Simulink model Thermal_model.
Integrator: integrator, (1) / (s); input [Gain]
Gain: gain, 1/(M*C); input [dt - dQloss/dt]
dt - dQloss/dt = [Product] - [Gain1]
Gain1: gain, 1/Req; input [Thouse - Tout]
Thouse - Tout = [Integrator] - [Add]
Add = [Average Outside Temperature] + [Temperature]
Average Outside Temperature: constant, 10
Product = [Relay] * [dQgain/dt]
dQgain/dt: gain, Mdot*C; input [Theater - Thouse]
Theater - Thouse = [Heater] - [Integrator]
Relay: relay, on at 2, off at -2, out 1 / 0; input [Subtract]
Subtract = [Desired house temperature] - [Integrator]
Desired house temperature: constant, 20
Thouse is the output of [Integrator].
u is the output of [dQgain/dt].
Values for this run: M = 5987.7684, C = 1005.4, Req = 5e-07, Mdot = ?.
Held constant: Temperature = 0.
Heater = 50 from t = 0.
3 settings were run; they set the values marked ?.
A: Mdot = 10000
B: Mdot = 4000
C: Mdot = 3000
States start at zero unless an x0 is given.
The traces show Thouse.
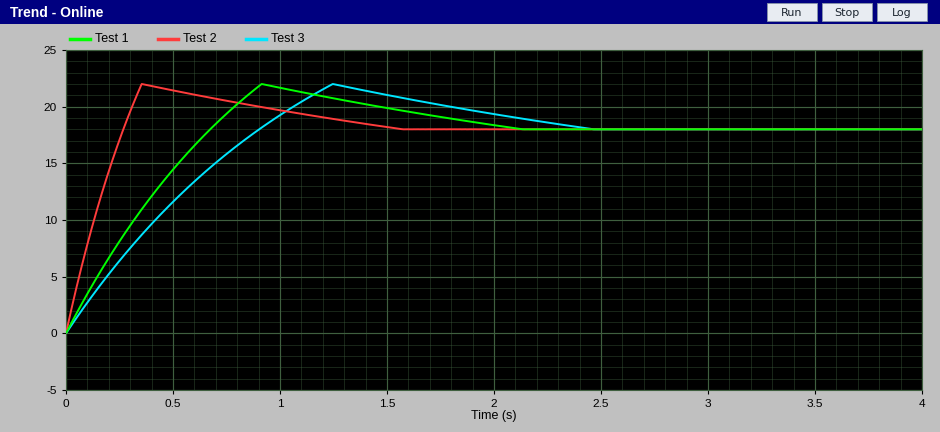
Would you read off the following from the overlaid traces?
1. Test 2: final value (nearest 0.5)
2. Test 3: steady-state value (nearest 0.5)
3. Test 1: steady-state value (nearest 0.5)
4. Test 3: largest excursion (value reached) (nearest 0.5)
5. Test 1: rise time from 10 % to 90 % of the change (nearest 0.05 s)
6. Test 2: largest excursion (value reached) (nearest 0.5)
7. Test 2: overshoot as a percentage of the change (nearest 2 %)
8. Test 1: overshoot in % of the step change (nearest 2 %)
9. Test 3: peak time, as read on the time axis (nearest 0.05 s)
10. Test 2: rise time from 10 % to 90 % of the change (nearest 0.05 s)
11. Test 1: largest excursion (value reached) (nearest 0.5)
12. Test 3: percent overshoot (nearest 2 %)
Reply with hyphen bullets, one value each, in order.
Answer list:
- 18.0
- 18.0
- 18.0
- 22.0
- 0.55 s
- 22.0
- 22 %
- 22 %
- 1.25 s
- 0.20 s
- 22.0
- 22 %
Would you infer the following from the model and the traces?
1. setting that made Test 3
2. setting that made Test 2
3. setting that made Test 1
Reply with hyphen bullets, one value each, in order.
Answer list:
- C
- A
- B
